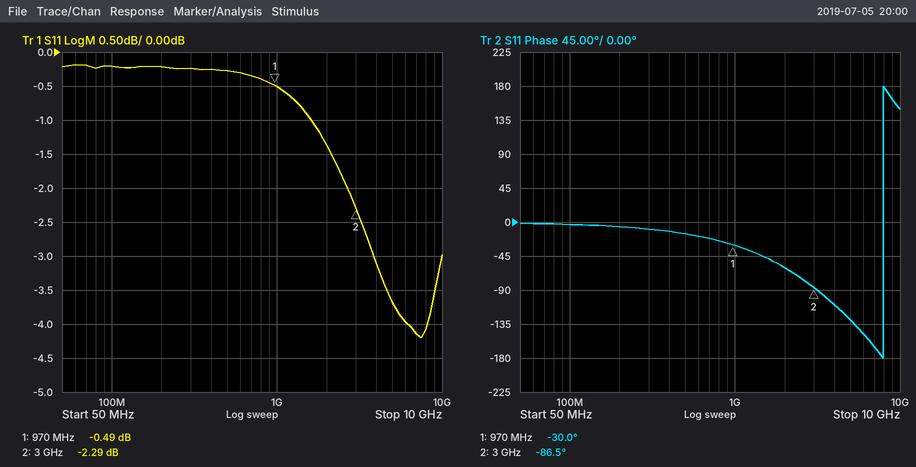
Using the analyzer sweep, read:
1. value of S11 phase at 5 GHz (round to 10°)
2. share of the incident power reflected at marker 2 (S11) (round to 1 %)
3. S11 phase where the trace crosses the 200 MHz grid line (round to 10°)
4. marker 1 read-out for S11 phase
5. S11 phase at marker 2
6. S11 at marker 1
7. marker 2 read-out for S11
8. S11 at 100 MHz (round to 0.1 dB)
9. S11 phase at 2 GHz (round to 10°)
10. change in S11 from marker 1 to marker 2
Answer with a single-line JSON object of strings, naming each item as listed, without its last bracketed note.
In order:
{"value of S11 phase at 5 GHz": "-130°", "share of the incident power reflected at marker 2 (S11)": "59 %", "S11 phase where the trace crosses the 200 MHz grid line": "-10°", "marker 1 read-out for S11 phase": "-30.0°", "S11 phase at marker 2": "-86.5°", "S11 at marker 1": "-0.49 dB", "marker 2 read-out for S11": "-2.29 dB", "S11 at 100 MHz": "-0.2 dB", "S11 phase at 2 GHz": "-60°", "change in S11 from marker 1 to marker 2": "-1.80 dB"}
